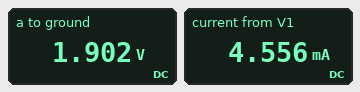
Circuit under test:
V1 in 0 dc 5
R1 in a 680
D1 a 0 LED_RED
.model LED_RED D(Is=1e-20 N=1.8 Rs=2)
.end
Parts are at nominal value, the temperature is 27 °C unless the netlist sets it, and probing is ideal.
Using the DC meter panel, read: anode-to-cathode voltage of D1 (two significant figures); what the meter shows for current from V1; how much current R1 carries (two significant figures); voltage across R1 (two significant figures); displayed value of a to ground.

1.9 V
4.556 mA
4.6 mA
3.1 V
1.902 V
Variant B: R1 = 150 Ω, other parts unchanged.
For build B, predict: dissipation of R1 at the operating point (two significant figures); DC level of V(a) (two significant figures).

60 mW
2.0 V
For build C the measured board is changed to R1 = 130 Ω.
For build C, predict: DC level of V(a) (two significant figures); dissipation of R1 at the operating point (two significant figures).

2.0 V
69 mW
